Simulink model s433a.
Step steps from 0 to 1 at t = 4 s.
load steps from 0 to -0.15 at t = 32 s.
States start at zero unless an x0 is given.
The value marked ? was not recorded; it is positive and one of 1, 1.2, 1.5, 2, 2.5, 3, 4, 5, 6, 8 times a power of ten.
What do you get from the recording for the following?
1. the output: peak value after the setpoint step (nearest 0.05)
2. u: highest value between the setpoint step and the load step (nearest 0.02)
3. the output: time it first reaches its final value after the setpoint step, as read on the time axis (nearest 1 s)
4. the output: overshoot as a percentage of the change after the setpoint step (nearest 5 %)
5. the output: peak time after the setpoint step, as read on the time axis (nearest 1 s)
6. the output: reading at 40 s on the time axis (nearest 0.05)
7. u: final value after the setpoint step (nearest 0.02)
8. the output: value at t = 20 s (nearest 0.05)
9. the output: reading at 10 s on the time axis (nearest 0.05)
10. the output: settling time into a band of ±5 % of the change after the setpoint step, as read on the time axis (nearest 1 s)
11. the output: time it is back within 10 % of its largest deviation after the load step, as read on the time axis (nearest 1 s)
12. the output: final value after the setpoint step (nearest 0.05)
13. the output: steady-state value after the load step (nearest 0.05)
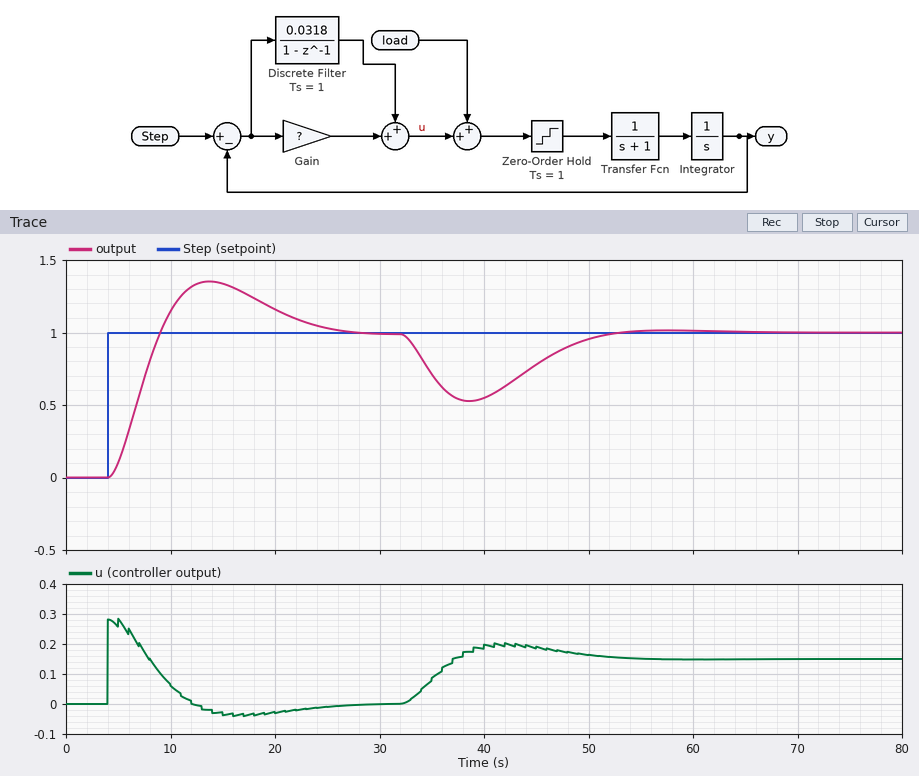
1.35
0.28
9 s
35 %
14 s
0.55
0.00
1.15
1.15
24 s
50 s
1.00
1.00
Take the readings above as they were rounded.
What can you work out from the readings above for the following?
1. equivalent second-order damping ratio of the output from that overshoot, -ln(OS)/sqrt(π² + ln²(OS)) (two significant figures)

0.32
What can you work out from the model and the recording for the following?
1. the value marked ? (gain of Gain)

0.25
